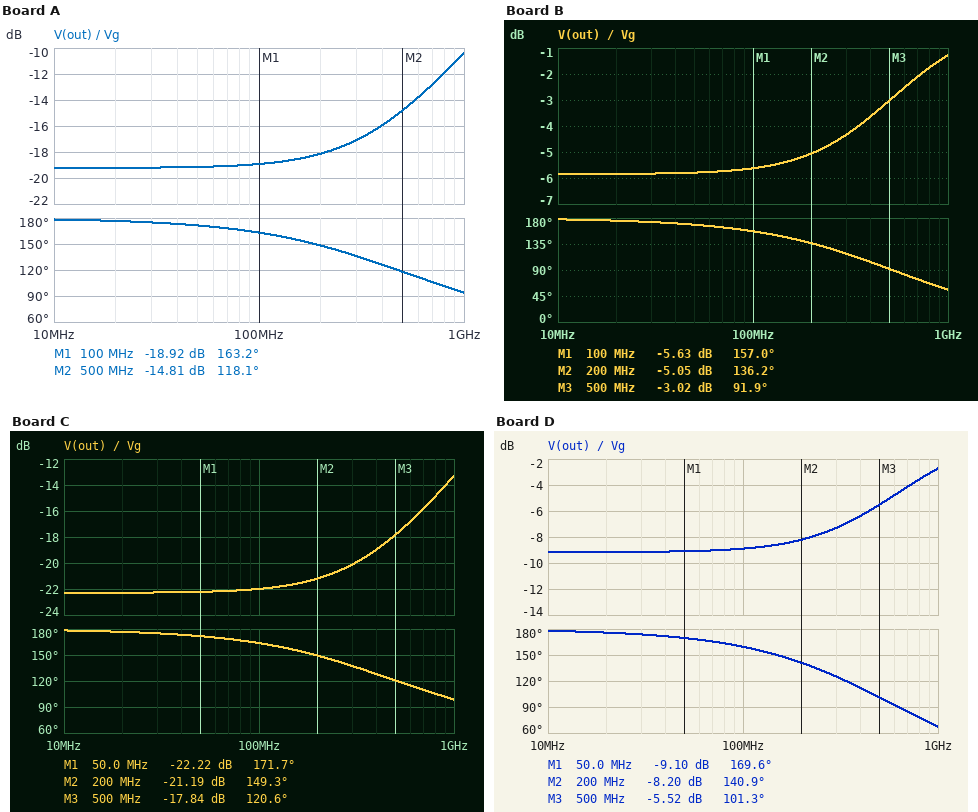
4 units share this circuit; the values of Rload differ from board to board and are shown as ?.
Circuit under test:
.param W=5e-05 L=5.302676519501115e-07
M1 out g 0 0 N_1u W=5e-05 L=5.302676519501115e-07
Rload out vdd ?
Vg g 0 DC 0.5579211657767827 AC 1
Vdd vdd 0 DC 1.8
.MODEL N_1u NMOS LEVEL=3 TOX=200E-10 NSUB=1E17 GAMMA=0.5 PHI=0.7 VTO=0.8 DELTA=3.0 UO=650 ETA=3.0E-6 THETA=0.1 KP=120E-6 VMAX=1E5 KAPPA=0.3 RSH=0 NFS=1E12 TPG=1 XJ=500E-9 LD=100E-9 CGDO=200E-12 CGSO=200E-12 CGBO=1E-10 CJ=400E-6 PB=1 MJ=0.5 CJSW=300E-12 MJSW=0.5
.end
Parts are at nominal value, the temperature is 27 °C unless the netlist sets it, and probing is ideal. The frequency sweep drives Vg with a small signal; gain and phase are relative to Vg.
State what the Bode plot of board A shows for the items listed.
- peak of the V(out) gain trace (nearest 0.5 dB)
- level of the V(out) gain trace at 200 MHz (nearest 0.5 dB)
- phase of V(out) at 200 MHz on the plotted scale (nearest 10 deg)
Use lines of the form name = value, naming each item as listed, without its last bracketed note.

peak of the V(out) gain trace = -10.5 dB
level of the V(out) gain trace at 200 MHz = -18.0 dB
phase of V(out) at 200 MHz on the plotted scale = 150 deg
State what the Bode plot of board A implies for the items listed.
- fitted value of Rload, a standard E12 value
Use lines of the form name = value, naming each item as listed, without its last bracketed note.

fitted value of Rload, a standard E12 value = 4.7 kΩ
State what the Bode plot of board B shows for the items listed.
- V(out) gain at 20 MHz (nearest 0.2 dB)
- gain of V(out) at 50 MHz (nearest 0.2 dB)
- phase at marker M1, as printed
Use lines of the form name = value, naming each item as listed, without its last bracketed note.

V(out) gain at 20 MHz = -5.8 dB
gain of V(out) at 50 MHz = -5.8 dB
phase at marker M1, as printed = 157.0 deg
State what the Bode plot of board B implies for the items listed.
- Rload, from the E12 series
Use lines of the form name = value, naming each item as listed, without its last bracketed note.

Rload, from the E12 series = 22 kΩ
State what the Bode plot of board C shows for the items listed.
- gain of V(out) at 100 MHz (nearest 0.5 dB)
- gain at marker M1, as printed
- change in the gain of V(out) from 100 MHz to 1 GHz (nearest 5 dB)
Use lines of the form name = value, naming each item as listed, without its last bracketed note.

gain of V(out) at 100 MHz = -22.0 dB
gain at marker M1, as printed = -22.22 dB
change in the gain of V(out) from 100 MHz to 1 GHz = 10 dB
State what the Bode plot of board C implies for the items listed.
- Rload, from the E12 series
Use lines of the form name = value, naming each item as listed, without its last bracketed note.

Rload, from the E12 series = 3.3 kΩ
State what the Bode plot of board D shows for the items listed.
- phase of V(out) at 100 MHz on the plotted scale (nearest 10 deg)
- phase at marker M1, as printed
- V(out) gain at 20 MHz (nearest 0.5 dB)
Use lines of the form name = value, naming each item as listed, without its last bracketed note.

phase of V(out) at 100 MHz on the plotted scale = 160 deg
phase at marker M1, as printed = 169.6 deg
V(out) gain at 20 MHz = -9.0 dB
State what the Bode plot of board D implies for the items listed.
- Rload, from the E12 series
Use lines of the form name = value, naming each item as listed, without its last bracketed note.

Rload, from the E12 series = 15 kΩ
